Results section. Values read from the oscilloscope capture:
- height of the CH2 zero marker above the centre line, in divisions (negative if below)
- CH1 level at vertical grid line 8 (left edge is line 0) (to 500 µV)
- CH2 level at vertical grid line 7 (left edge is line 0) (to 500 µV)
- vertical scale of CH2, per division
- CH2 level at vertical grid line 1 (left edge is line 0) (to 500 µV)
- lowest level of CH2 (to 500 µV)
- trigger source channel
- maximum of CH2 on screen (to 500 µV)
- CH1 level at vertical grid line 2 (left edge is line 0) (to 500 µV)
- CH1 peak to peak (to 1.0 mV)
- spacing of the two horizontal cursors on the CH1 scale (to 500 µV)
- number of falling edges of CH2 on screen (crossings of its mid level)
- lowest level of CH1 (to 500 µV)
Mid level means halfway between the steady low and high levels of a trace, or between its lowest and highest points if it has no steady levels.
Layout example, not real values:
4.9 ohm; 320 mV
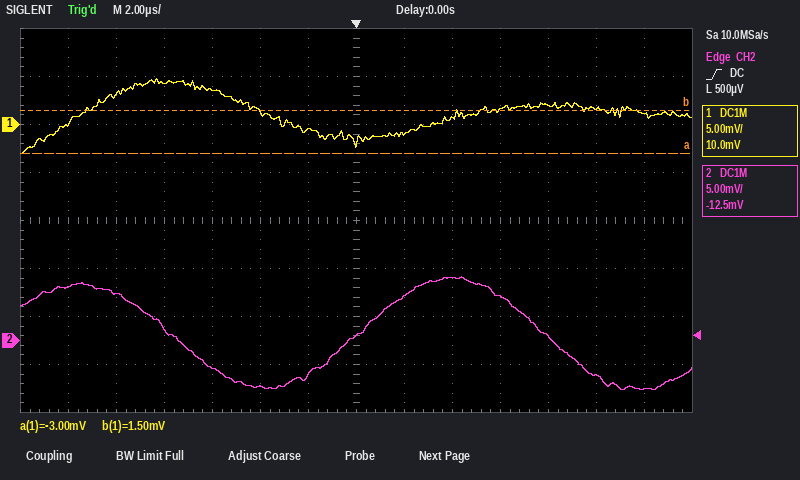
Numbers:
-2.5 div; -1.0 mV; 500 µV; 5 mV; 5.5 mV; -5.0 mV; CH2; 6.5 mV; 3.0 mV; 8.0 mV; 4.5 mV; 2; -3.0 mV
